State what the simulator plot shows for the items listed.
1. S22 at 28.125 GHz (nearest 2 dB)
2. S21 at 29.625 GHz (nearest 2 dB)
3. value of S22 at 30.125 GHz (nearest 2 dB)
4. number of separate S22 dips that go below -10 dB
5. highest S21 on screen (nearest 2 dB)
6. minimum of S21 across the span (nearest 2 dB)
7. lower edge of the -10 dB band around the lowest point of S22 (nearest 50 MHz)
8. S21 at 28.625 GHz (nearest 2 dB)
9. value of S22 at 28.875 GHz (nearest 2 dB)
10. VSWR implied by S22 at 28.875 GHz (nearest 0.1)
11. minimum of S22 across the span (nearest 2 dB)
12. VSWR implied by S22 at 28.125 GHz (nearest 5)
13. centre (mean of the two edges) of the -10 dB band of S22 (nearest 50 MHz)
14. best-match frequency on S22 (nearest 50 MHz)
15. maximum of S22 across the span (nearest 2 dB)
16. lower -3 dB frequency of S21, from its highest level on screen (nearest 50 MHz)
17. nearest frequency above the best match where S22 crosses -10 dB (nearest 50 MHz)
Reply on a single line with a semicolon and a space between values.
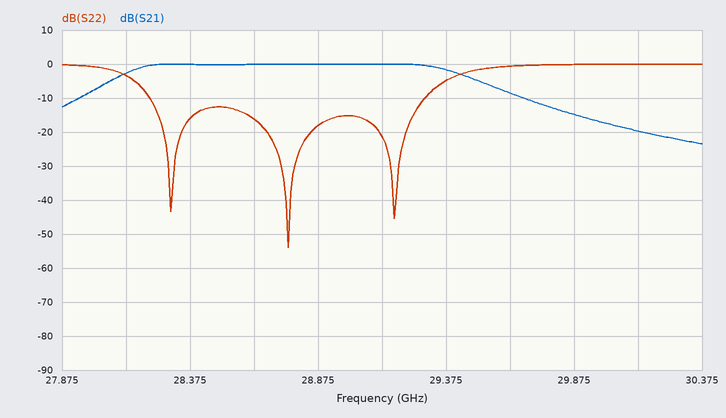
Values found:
-4 dB; -8 dB; 0 dB; 3; 0 dB; -24 dB; 28.20 GHz; 0 dB; -18 dB; 1.3; -54 dB; 5; 28.75 GHz; 28.75 GHz; 0 dB; 28.10 GHz; 29.30 GHz
